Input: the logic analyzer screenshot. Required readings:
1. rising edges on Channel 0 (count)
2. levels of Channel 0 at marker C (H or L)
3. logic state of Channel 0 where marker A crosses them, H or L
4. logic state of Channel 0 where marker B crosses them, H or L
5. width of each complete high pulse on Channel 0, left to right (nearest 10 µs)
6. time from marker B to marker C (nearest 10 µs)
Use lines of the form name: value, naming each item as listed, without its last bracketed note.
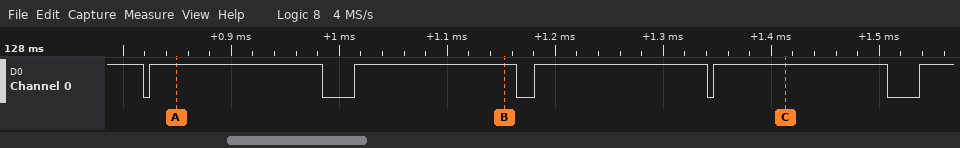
rising edges on Channel 0: 5
levels of Channel 0 at marker C: Channel 0=H
logic state of Channel 0 where marker A crosses them, H or L: Channel 0=H
logic state of Channel 0 where marker B crosses them, H or L: Channel 0=H
width of each complete high pulse on Channel 0, left to right: 160 µs, 150 µs, 160 µs, 160 µs
time from marker B to marker C: 260 µs
